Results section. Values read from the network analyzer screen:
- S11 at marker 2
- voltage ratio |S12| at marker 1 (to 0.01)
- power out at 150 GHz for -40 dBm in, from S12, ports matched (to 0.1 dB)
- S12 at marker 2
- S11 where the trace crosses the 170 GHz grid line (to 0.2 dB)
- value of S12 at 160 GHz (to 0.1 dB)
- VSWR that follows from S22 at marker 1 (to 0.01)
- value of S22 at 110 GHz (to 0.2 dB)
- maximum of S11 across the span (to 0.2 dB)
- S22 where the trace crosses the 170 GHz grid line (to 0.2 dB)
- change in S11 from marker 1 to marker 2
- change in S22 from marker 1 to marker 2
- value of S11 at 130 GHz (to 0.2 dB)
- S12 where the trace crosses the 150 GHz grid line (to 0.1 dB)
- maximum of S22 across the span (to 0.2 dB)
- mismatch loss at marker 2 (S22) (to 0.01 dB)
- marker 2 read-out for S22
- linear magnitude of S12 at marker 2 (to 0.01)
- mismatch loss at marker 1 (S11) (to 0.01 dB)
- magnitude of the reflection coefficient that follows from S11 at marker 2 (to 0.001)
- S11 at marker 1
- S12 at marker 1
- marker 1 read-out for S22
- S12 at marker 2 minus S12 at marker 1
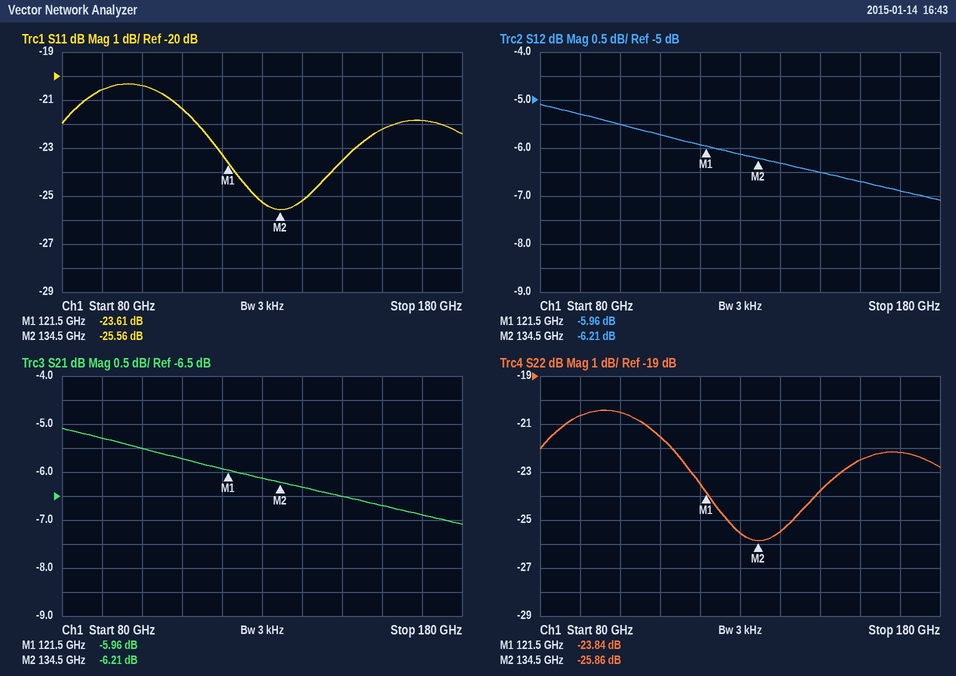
-25.56 dB
0.50
-46.5 dBm
-6.21 dB
-21.8 dB
-6.7 dB
1.14
-21.6 dB
-20.4 dB
-22.2 dB
-1.95 dB
-2.02 dB
-25.2 dB
-6.5 dB
-20.4 dB
0.01 dB
-25.86 dB
0.49
0.02 dB
0.053
-23.61 dB
-5.96 dB
-23.84 dB
-0.25 dB
